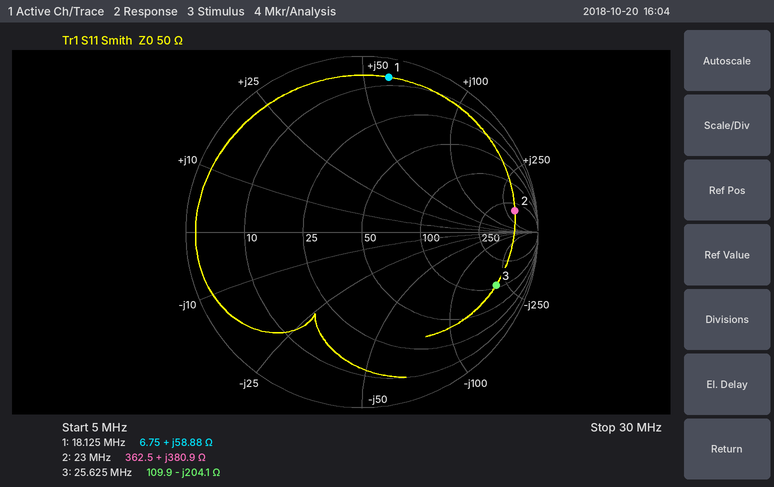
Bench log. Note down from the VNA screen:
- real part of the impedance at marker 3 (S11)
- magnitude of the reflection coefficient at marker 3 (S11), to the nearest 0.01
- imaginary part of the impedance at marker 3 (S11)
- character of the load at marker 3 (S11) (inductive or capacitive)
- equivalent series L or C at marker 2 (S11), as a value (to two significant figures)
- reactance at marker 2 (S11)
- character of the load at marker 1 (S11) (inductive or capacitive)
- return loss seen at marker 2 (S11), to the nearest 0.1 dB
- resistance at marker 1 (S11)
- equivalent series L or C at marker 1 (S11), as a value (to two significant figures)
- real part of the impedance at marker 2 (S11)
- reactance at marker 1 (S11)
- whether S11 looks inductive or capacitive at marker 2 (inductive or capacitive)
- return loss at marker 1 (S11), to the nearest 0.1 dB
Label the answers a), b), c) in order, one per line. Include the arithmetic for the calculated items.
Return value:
a) 109.9 Ω
b) 0.82
c) -204.1 Ω
d) capacitive
e) L = 380.9 Ω/(2π × 23 MHz) ≈ 2.6 µH
f) +380.9 Ω
g) inductive
h) 1.1 dB
i) 6.75 Ω
j) L = 58.88 Ω/(2π × 18.125 MHz) ≈ 517 nH, so 520 nH to two significant figures
k) 362.5 Ω
l) +58.88 Ω
m) inductive
n) 1.0 dB
